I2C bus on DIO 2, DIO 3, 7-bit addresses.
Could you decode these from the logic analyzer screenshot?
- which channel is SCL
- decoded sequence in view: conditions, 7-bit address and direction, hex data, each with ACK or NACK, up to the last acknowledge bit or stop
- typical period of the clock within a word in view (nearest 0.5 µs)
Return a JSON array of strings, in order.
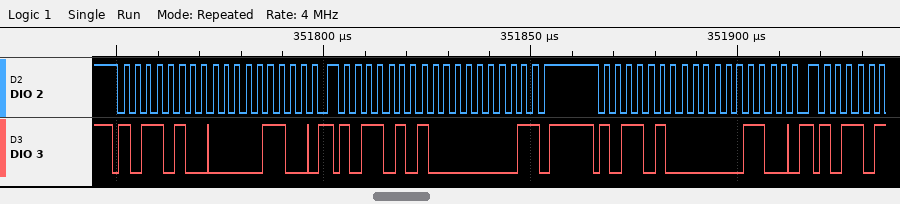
["DIO 2", "start, address 5A write ACK, 0C ACK, repeated start, address 5A read ACK, 01 NACK, stop, start, address 5A write ACK, 0C ACK", "2.5 µs"]
